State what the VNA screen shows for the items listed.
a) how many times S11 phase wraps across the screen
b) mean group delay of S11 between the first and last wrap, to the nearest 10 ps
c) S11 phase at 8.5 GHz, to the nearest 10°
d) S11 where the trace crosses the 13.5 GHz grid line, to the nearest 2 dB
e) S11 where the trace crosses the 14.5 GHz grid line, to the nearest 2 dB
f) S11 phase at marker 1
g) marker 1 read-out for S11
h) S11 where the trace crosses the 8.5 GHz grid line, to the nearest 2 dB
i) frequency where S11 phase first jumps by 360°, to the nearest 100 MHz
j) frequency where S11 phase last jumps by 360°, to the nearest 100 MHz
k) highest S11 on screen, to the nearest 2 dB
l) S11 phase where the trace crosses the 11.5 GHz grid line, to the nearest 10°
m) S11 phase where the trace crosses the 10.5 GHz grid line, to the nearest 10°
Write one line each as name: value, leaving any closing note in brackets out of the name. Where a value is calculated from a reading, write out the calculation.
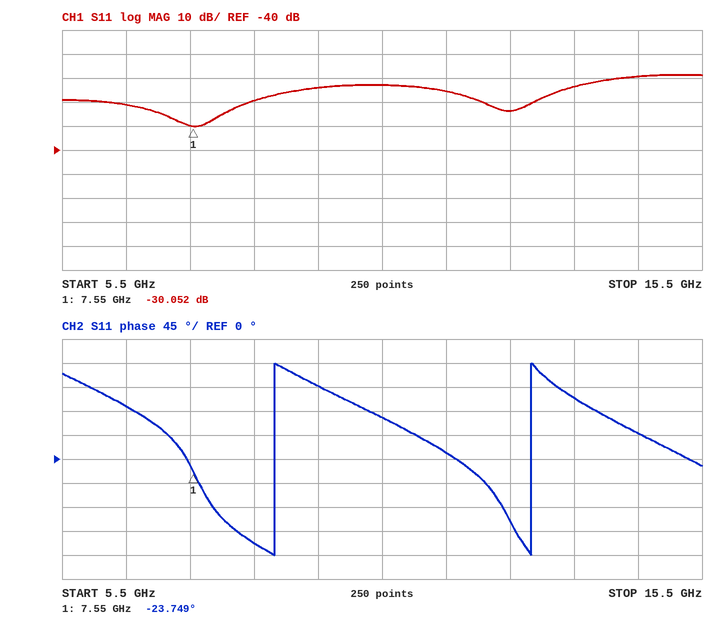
how many times S11 phase wraps across the screen: 2
mean group delay of S11 between the first and last wrap, to the nearest 10 ps: 1 cycle / (12.8 GHz − 8.8 GHz) ≈ 250 ps
S11 phase at 8.5 GHz, to the nearest 10°: -160°
S11 where the trace crosses the 13.5 GHz grid line, to the nearest 2 dB: -14 dB
S11 where the trace crosses the 14.5 GHz grid line, to the nearest 2 dB: -10 dB
S11 phase at marker 1: -23.749°
marker 1 read-out for S11: -30.052 dB
S11 where the trace crosses the 8.5 GHz grid line, to the nearest 2 dB: -20 dB
frequency where S11 phase first jumps by 360°, to the nearest 100 MHz: 8.8 GHz
frequency where S11 phase last jumps by 360°, to the nearest 100 MHz: 12.8 GHz
highest S11 on screen, to the nearest 2 dB: -8 dB
S11 phase where the trace crosses the 11.5 GHz grid line, to the nearest 10°: 10°
S11 phase where the trace crosses the 10.5 GHz grid line, to the nearest 10°: 80°
